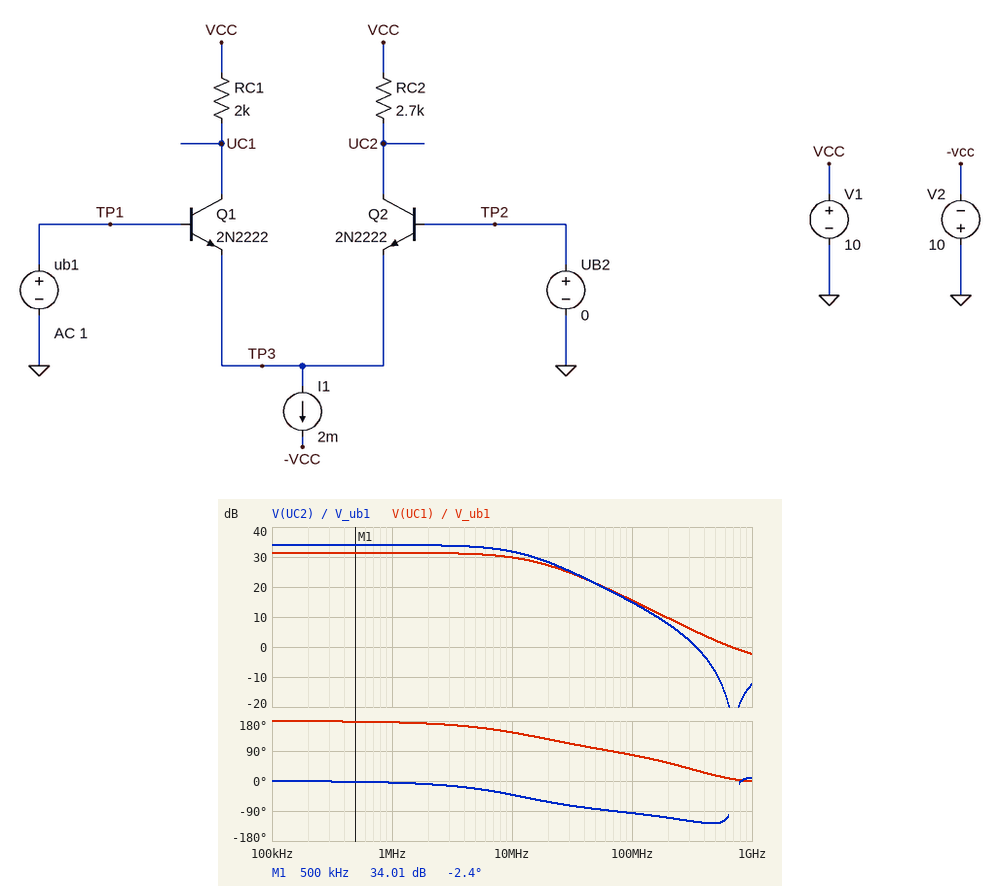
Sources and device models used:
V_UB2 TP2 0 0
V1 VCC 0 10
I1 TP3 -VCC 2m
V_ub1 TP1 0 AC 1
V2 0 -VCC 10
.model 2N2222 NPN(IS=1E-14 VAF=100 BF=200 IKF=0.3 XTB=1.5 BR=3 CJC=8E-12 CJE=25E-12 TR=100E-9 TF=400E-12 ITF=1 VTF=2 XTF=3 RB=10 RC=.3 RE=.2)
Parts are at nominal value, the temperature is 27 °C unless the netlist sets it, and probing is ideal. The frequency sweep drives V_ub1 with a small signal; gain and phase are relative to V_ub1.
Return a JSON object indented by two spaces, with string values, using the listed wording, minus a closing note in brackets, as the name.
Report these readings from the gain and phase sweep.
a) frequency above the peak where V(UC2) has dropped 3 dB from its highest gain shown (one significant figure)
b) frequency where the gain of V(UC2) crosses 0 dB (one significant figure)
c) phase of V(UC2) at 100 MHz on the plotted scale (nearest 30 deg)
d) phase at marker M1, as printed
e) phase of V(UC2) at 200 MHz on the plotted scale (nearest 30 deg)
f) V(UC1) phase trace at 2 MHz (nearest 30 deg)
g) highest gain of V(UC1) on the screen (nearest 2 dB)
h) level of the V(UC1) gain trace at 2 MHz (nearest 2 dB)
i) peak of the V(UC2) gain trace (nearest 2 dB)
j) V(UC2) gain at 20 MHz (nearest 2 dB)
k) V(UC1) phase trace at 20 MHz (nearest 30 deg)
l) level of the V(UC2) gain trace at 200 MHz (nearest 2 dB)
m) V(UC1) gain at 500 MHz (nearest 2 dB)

{
  "frequency above the peak where V(UC2) has dropped 3 dB from its highest gain shown": "10 MHz",
  "frequency where the gain of V(UC2) crosses 0 dB": "300 MHz",
  "phase of V(UC2) at 100 MHz on the plotted scale": "-90 deg",
  "phase at marker M1, as printed": "-2.4 deg",
  "phase of V(UC2) at 200 MHz on the plotted scale": "-120 deg",
  "V(UC1) phase trace at 2 MHz": "180 deg",
  "highest gain of V(UC1) on the screen": "32 dB",
  "level of the V(UC1) gain trace at 2 MHz": "32 dB",
  "peak of the V(UC2) gain trace": "34 dB",
  "V(UC2) gain at 20 MHz": "28 dB",
  "V(UC1) phase trace at 20 MHz": "120 deg",
  "level of the V(UC2) gain trace at 200 MHz": "8 dB",
  "V(UC1) gain at 500 MHz": "2 dB"
}
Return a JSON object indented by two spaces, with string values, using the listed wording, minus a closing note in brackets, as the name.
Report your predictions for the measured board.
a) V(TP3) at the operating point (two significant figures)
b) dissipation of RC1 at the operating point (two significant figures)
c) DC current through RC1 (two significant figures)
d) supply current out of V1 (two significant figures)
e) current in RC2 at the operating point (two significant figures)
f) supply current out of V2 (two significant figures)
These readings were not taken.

{
  "V(TP3) at the operating point": "-650 mV",
  "dissipation of RC1 at the operating point": "2.0 mW",
  "DC current through RC1": "1.0 mA",
  "supply current out of V1": "2.0 mA",
  "current in RC2 at the operating point": "990 µA",
  "supply current out of V2": "2.0 mA"
}
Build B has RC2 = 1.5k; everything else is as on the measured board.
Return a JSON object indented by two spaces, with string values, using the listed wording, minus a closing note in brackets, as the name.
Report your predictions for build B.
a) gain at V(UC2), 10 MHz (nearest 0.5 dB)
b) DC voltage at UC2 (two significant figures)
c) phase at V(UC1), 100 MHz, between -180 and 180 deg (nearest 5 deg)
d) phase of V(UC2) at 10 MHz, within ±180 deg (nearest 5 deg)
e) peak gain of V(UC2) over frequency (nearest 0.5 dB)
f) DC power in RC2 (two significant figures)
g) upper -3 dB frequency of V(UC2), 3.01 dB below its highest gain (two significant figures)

{
  "gain at V(UC2), 10 MHz": "28.0 dB",
  "DC voltage at UC2": "8.5 V",
  "phase at V(UC1), 100 MHz, between -180 and 180 deg": "75 deg",
  "phase of V(UC2) at 10 MHz, within ±180 deg": "-25 deg",
  "peak gain of V(UC2) over frequency": "29.0 dB",
  "DC power in RC2": "1.5 mW",
  "upper -3 dB frequency of V(UC2), 3.01 dB below its highest gain": "21 MHz"
}
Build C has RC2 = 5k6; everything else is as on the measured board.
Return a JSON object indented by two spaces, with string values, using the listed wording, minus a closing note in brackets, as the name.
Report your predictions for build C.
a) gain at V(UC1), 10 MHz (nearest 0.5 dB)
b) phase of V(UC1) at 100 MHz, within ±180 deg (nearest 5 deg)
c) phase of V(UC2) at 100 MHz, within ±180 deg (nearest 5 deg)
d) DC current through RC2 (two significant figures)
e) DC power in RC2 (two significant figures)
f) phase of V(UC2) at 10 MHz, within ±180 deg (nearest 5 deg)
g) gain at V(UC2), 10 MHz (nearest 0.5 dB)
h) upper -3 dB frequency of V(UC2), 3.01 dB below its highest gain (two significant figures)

{
  "gain at V(UC1), 10 MHz": "29.5 dB",
  "phase of V(UC1) at 100 MHz, within ±180 deg": "80 deg",
  "phase of V(UC2) at 100 MHz, within ±180 deg": "-100 deg",
  "DC current through RC2": "980 µA",
  "DC power in RC2": "5.4 mW",
  "phase of V(UC2) at 10 MHz, within ±180 deg": "-65 deg",
  "gain at V(UC2), 10 MHz": "34.0 dB",
  "upper -3 dB frequency of V(UC2), 3.01 dB below its highest gain": "5.6 MHz"
}
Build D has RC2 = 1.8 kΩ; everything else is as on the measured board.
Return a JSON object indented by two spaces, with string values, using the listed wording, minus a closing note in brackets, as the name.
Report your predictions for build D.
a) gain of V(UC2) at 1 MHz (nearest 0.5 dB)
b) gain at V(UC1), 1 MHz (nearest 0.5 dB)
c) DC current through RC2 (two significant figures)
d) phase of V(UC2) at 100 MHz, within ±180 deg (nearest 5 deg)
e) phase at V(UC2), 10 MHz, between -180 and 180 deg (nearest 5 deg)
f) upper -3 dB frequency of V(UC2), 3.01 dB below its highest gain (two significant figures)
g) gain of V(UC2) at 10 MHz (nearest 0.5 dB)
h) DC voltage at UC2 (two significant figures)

{
  "gain of V(UC2) at 1 MHz": "30.5 dB",
  "gain at V(UC1), 1 MHz": "31.5 dB",
  "DC current through RC2": "1.0 mA",
  "phase of V(UC2) at 100 MHz, within ±180 deg": "-90 deg",
  "phase at V(UC2), 10 MHz, between -180 and 180 deg": "-30 deg",
  "upper -3 dB frequency of V(UC2), 3.01 dB below its highest gain": "18 MHz",
  "gain of V(UC2) at 10 MHz": "29.5 dB",
  "DC voltage at UC2": "8.2 V"
}
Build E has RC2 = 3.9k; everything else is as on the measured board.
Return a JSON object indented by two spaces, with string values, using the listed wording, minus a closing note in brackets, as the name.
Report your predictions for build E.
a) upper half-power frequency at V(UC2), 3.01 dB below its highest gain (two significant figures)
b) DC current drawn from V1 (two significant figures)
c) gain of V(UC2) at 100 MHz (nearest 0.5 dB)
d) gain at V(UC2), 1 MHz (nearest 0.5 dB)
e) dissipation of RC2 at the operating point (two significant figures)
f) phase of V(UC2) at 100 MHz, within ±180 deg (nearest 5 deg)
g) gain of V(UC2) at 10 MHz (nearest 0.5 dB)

{
  "upper half-power frequency at V(UC2), 3.01 dB below its highest gain": "8.5 MHz",
  "DC current drawn from V1": "2.0 mA",
  "gain of V(UC2) at 100 MHz": "14.5 dB",
  "gain at V(UC2), 1 MHz": "37.0 dB",
  "dissipation of RC2 at the operating point": "3.8 mW",
  "phase of V(UC2) at 100 MHz, within ±180 deg": "-100 deg",
  "gain of V(UC2) at 10 MHz": "33.5 dB"
}
